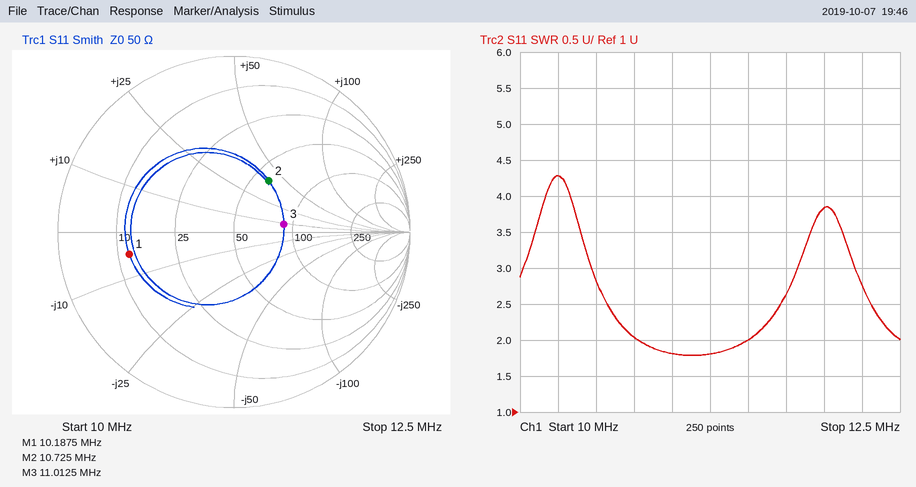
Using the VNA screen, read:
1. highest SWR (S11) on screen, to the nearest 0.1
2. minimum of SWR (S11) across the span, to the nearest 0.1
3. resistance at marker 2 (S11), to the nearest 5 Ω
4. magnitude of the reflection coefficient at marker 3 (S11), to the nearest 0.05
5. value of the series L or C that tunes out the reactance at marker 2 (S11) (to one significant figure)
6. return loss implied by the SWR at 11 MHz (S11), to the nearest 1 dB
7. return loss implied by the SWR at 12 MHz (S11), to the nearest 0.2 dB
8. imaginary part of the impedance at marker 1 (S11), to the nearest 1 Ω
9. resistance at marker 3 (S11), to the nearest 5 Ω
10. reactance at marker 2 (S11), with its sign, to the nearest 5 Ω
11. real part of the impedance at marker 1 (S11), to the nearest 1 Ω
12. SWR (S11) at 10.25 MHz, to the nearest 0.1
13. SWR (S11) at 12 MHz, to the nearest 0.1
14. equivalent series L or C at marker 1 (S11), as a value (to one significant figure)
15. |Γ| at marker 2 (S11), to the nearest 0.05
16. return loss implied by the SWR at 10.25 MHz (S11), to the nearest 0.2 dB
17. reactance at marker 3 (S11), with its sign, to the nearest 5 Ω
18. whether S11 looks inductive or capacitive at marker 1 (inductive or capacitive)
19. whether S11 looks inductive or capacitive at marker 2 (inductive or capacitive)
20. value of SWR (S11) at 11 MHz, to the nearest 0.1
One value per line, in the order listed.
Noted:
4.3
1.8
60 Ω
0.30
400 pF
11 dB
4.6 dB
-5 Ω
90 Ω
+40 Ω
12 Ω
4.3
3.8
3 nF
0.35
4.2 dB
+10 Ω
capacitive
inductive
1.8
